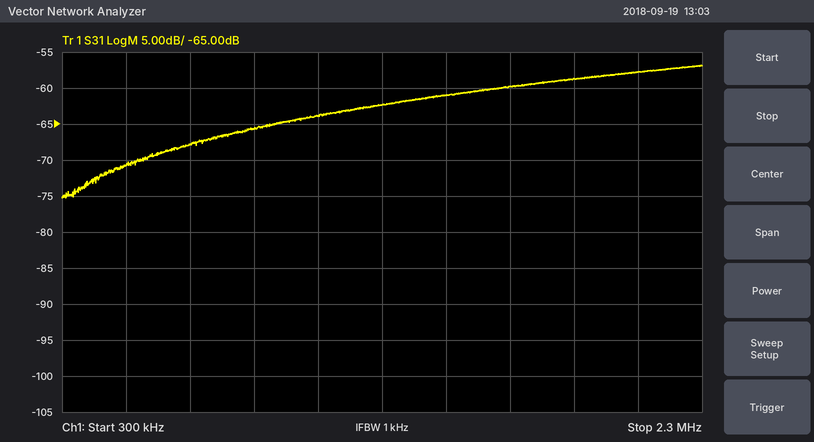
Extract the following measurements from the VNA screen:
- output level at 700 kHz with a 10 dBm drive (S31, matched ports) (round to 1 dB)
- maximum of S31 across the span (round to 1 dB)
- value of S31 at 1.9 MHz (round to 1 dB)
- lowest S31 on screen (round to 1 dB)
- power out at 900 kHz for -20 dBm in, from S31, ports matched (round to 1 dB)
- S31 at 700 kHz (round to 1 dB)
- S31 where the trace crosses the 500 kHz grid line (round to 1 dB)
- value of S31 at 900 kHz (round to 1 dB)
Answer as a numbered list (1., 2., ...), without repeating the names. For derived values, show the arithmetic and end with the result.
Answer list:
1. 10 dBm + (-68 dB) = -58 dBm
2. -57 dB
3. -59 dB
4. -75 dB
5. -20 dBm + (-66 dB) = -86 dBm
6. -68 dB
7. -71 dB
8. -66 dB
